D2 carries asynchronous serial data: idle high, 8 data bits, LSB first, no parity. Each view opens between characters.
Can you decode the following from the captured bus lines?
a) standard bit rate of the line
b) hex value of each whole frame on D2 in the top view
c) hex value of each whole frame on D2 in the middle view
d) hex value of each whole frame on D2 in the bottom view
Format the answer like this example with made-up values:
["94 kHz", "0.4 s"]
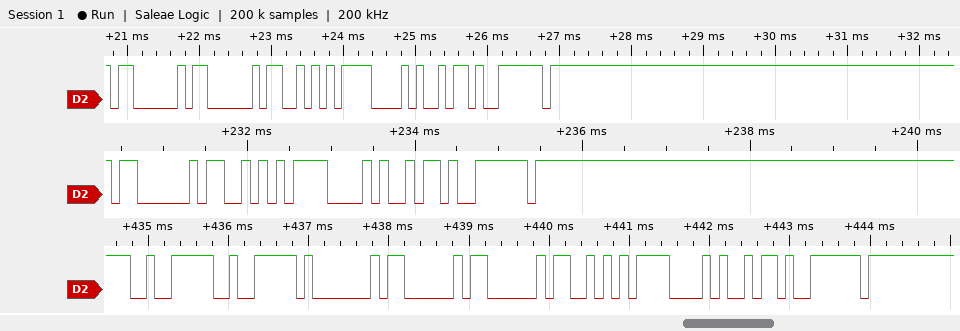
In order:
["9600 baud", "03, 03, 53, 0F, 69, 7E", "03, 53, 0F, 69, 7E", "F2, F2, 01, 03, 03, 53, 0F, 69, 7E"]
